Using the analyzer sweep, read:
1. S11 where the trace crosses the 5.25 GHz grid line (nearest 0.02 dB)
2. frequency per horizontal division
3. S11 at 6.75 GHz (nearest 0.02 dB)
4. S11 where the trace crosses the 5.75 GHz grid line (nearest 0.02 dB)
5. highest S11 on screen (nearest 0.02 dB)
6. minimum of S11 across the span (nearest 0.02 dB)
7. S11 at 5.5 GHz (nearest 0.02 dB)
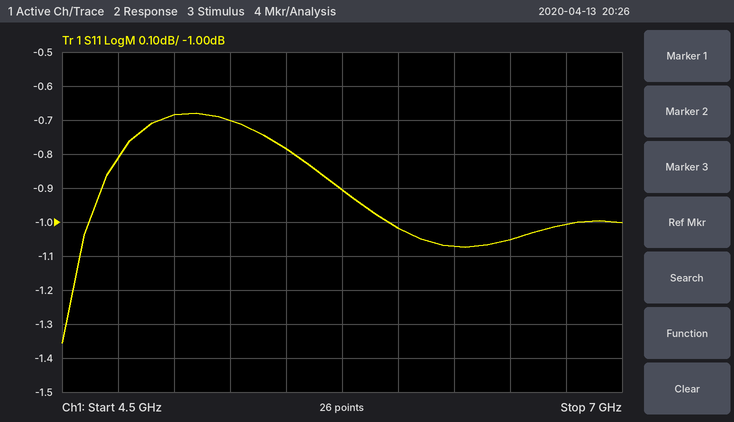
-0.70 dB
250 MHz
-1.00 dB
-0.90 dB
-0.68 dB
-1.36 dB
-0.78 dB
